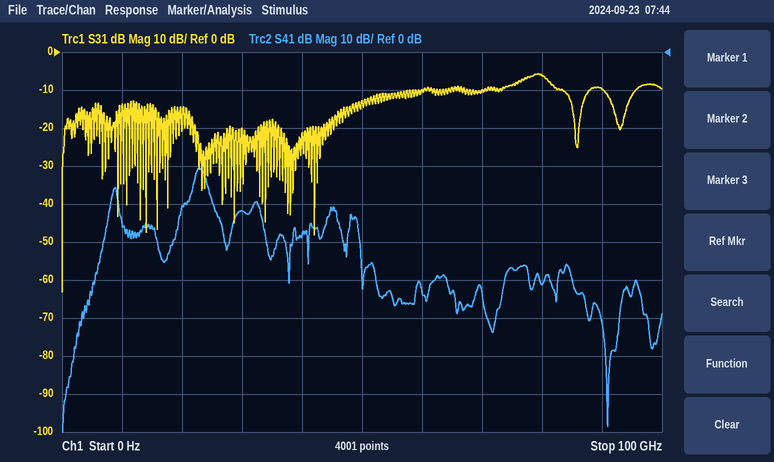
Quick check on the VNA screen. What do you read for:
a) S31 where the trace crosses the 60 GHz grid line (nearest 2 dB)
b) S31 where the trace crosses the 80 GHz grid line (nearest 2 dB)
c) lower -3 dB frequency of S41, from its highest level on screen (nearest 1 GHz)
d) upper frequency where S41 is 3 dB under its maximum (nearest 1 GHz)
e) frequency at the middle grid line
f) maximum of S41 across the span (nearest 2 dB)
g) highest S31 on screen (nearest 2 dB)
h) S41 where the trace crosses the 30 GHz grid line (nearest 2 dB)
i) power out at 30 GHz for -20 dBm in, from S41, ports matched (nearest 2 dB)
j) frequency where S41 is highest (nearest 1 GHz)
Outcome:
-10 dB
-6 dB
22 GHz
24 GHz
50 GHz
-30 dB
-6 dB
-42 dB
-62 dBm
23 GHz
